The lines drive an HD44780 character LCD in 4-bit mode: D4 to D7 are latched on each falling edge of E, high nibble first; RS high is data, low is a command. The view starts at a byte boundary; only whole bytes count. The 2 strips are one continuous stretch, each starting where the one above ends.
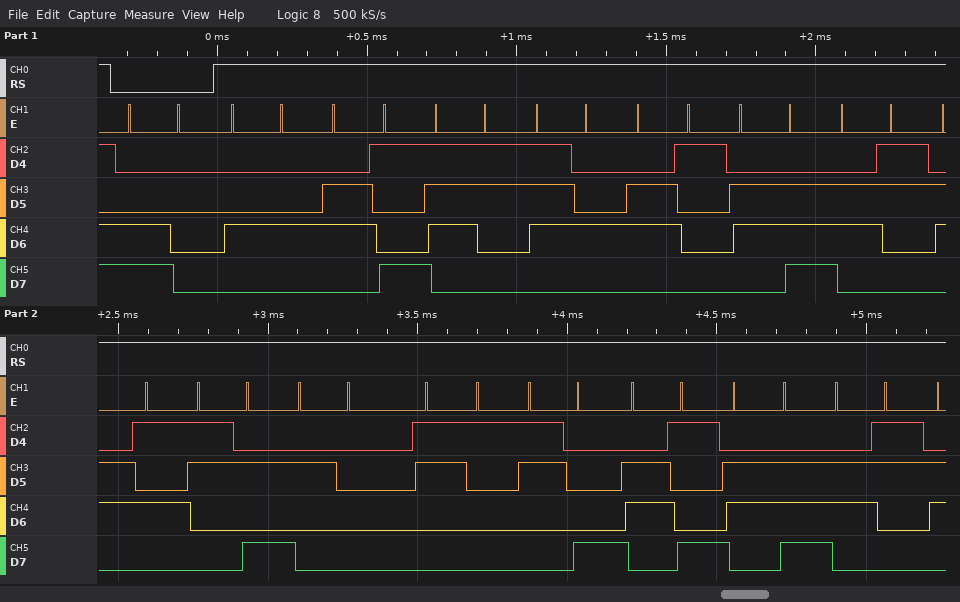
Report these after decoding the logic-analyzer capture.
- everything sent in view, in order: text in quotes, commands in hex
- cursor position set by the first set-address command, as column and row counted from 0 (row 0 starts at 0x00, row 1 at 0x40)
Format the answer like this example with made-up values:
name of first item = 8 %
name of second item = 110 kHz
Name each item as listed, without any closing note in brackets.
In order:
everything sent in view, in order: text in quotes, commands in hex = 0xC0 "Distance: 18inc"
cursor position set by the first set-address command, as column and row counted from 0 = column 0, row 1
